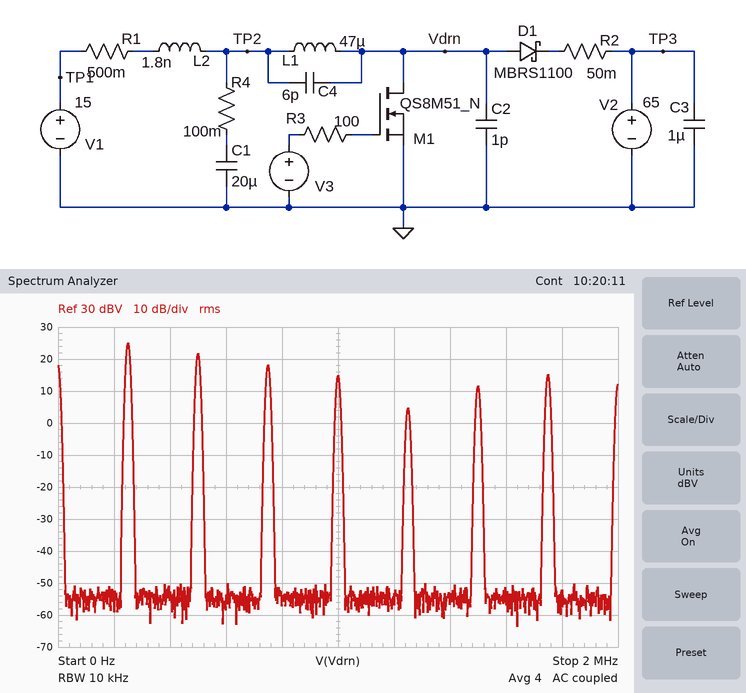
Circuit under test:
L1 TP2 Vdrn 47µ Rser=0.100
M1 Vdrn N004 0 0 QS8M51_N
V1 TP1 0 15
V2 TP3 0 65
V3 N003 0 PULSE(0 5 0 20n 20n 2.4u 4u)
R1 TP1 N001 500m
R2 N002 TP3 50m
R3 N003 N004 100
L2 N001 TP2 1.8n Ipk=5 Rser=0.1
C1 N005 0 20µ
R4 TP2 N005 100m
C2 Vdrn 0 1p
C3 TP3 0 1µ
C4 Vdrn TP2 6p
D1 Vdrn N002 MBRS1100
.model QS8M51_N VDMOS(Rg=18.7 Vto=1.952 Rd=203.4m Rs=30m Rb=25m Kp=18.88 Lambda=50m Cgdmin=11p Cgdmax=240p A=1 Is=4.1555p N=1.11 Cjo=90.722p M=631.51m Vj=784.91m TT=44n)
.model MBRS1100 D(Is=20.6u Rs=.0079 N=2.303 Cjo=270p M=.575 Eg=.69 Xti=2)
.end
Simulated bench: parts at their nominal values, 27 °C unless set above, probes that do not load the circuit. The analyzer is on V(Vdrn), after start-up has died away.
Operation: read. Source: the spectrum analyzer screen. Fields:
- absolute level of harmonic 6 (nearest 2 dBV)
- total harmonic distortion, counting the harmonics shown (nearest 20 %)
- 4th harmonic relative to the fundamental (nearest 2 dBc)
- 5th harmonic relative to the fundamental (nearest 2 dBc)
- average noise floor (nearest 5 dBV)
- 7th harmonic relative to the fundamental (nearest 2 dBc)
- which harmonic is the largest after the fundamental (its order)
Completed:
12 dBV
100 %
-10 dBc
-20 dBc
-55 dBV
-10 dBc
2
